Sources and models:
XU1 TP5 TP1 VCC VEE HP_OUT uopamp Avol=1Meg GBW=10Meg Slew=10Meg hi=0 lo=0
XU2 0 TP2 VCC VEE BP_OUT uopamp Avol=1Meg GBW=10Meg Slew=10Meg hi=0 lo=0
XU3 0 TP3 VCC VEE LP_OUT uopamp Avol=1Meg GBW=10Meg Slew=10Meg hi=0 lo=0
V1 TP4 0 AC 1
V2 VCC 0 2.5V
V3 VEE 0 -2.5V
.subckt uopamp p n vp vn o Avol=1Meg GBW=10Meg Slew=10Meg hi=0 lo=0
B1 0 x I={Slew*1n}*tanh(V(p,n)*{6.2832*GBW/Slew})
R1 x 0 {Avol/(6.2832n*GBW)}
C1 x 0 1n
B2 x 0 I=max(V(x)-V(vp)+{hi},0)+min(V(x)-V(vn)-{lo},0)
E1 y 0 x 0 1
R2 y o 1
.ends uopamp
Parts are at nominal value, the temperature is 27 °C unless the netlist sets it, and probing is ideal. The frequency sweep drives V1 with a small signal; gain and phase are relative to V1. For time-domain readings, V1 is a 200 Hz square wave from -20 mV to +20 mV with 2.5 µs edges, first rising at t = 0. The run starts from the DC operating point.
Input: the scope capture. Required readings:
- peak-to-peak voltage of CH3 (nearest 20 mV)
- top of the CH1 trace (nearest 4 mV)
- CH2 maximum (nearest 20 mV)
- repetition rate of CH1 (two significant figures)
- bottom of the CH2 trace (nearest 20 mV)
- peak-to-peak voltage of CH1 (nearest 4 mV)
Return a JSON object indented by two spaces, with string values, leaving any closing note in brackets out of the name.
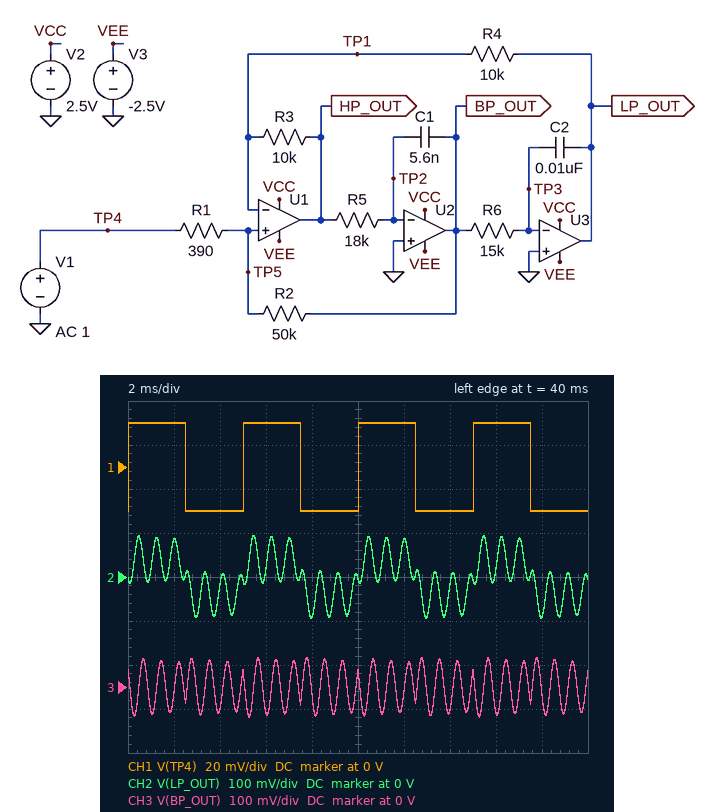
{
  "peak-to-peak voltage of CH3": "140 mV",
  "top of the CH1 trace": "20 mV",
  "CH2 maximum": "100 mV",
  "repetition rate of CH1": "200 Hz",
  "bottom of the CH2 trace": "-100 mV",
  "peak-to-peak voltage of CH1": "40 mV"
}
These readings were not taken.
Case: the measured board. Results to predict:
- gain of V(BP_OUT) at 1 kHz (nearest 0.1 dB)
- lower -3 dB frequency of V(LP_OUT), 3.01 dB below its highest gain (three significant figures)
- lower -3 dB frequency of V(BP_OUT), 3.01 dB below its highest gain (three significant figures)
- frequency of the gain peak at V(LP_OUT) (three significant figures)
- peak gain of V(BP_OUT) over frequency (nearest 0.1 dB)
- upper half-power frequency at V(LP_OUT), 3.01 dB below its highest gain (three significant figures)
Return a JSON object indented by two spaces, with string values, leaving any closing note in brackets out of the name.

{
  "gain of V(BP_OUT) at 1 kHz": "13.3 dB",
  "lower -3 dB frequency of V(LP_OUT), 3.01 dB below its highest gain": "1.28 kHz",
  "lower -3 dB frequency of V(BP_OUT), 3.01 dB below its highest gain": "1.28 kHz",
  "frequency of the gain peak at V(LP_OUT)": "1.29 kHz",
  "peak gain of V(BP_OUT) over frequency": "42.4 dB",
  "upper half-power frequency at V(LP_OUT), 3.01 dB below its highest gain": "1.31 kHz"
}
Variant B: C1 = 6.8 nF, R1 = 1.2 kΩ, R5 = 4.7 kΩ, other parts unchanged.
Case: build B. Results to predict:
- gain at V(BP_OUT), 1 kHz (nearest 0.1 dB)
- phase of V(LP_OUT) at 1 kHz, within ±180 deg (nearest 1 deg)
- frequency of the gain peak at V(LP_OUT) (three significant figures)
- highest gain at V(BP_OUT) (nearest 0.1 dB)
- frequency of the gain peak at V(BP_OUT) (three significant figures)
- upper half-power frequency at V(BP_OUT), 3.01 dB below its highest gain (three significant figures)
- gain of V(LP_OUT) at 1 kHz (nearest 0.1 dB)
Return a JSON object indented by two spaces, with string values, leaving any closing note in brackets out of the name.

{
  "gain at V(BP_OUT), 1 kHz": "7.1 dB",
  "phase of V(LP_OUT) at 1 kHz, within ±180 deg": "-3 deg",
  "frequency of the gain peak at V(LP_OUT)": "2.29 kHz",
  "highest gain at V(BP_OUT)": "32.5 dB",
  "frequency of the gain peak at V(BP_OUT)": "2.30 kHz",
  "upper half-power frequency at V(BP_OUT), 3.01 dB below its highest gain": "2.42 kHz",
  "gain of V(LP_OUT) at 1 kHz": "7.6 dB"
}
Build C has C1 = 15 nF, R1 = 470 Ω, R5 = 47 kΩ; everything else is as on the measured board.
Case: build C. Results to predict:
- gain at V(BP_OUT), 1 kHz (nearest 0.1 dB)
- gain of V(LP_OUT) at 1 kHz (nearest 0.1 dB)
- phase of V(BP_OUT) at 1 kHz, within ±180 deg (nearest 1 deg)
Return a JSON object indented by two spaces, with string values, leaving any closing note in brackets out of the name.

{
  "gain at V(BP_OUT), 1 kHz": "-4.6 dB",
  "gain of V(LP_OUT) at 1 kHz": "-4.1 dB",
  "phase of V(BP_OUT) at 1 kHz, within ±180 deg": "90 deg"
}
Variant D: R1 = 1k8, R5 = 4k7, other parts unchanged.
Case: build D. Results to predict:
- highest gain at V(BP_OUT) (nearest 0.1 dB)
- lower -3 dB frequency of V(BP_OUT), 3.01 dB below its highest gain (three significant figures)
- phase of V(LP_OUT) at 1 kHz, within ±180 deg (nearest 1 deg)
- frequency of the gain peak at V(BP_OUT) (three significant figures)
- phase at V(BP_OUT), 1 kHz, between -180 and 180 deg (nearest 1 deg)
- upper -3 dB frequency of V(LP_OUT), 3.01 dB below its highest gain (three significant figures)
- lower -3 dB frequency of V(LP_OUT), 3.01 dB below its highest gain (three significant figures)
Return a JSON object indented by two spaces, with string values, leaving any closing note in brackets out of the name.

{
  "highest gain at V(BP_OUT)": "28.9 dB",
  "lower -3 dB frequency of V(BP_OUT), 3.01 dB below its highest gain": "2.33 kHz",
  "phase of V(LP_OUT) at 1 kHz, within ±180 deg": "-4 deg",
  "frequency of the gain peak at V(BP_OUT)": "2.53 kHz",
  "phase at V(BP_OUT), 1 kHz, between -180 and 180 deg": "-94 deg",
  "upper -3 dB frequency of V(LP_OUT), 3.01 dB below its highest gain": "2.72 kHz",
  "lower -3 dB frequency of V(LP_OUT), 3.01 dB below its highest gain": "2.30 kHz"
}
